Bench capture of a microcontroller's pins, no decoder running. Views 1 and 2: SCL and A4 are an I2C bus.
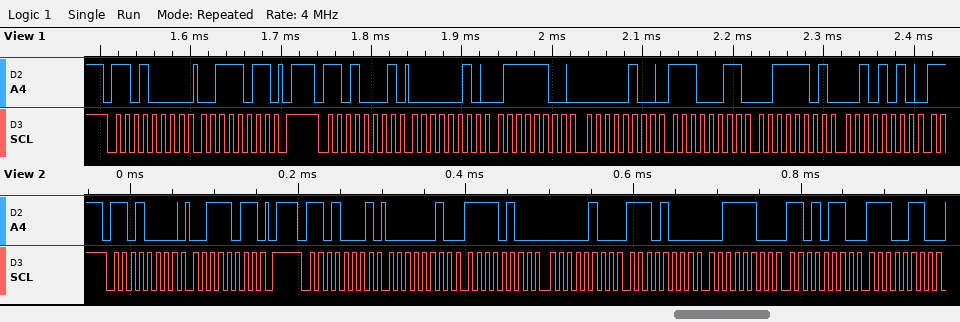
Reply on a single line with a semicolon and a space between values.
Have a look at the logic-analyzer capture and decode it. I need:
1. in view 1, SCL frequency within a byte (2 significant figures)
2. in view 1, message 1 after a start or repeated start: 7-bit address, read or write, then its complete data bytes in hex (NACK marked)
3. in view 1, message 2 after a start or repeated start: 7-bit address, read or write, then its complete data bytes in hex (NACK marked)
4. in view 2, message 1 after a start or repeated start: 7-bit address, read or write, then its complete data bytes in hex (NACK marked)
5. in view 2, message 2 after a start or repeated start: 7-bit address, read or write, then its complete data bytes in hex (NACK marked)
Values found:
100 kHz; 0x68 write: 3B; 0x68 read: 02 7C 04 E3 3D 2A; 0x68 write: 3B; 0x68 read: 02 F4 04 E8 3C D6 E6
